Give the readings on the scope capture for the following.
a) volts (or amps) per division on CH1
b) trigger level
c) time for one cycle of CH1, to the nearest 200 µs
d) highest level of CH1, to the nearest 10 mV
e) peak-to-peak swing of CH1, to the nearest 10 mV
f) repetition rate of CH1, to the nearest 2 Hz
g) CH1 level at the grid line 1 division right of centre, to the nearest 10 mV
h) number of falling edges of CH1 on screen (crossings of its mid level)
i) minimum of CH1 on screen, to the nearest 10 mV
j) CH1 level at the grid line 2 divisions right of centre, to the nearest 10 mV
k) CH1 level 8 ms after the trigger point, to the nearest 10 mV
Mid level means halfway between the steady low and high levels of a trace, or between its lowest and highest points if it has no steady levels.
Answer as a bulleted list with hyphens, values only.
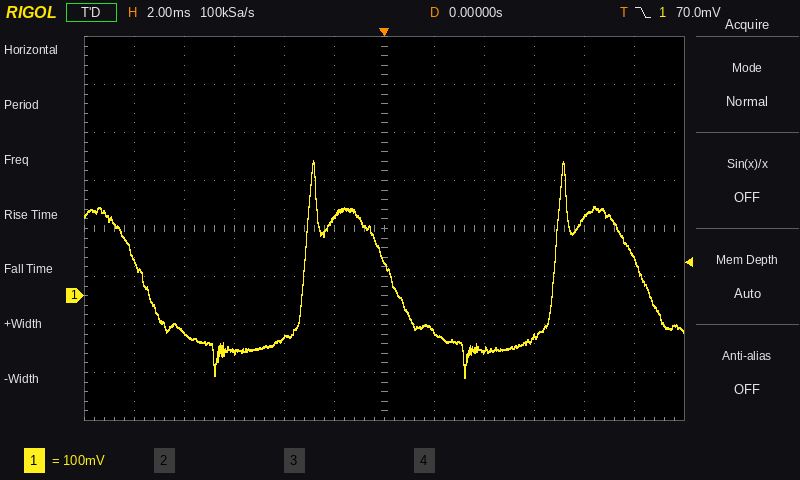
- 100 mV
- 70.0 mV
- 10.0 ms
- 280 mV
- 450 mV
- 100 Hz
- -80 mV
- 3
- -170 mV
- -110 mV
- 160 mV
